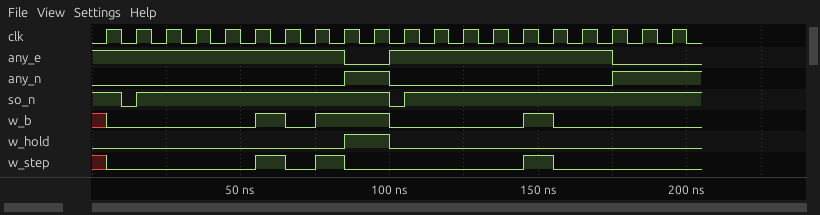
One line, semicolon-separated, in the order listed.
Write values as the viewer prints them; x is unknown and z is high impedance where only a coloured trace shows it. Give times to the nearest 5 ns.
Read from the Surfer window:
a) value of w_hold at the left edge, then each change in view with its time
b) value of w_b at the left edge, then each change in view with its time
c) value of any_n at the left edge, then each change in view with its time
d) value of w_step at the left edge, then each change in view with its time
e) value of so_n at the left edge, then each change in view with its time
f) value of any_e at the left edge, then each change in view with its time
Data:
0, 1 at 85 ns, 0 at 100 ns; x, 0 at 5 ns, 1 at 55 ns, 0 at 65 ns, 1 at 75 ns, 0 at 100 ns, 1 at 145 ns, 0 at 155 ns; 0, 1 at 85 ns, 0 at 100 ns, 1 at 175 ns; x, 0 at 5 ns, 1 at 55 ns, 0 at 65 ns, 1 at 75 ns, 0 at 85 ns, 1 at 145 ns, 0 at 155 ns; 1, 0 at 10 ns, 1 at 15 ns, 0 at 100 ns, 1 at 105 ns; 1, 0 at 85 ns, 1 at 100 ns, 0 at 175 ns
